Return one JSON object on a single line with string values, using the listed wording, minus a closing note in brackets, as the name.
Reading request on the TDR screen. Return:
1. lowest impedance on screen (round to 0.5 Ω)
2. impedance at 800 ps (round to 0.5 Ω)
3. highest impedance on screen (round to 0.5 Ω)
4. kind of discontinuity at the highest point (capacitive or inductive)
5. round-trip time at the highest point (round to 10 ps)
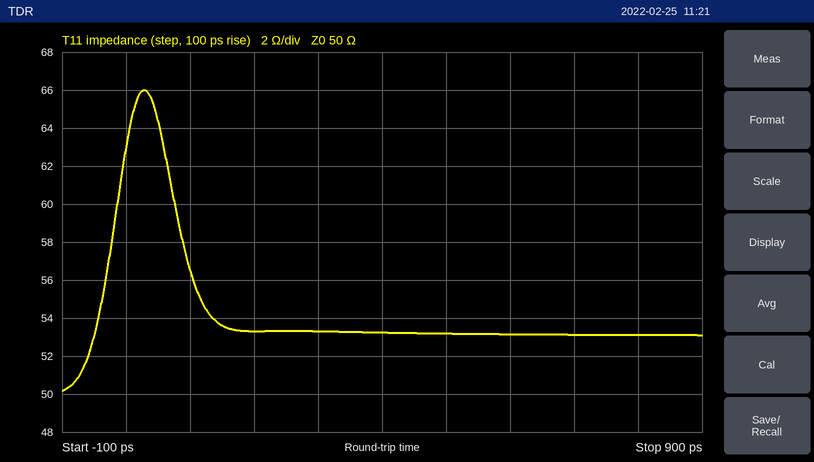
{"lowest impedance on screen": "50.0 Ω", "impedance at 800 ps": "53.0 Ω", "highest impedance on screen": "66.0 Ω", "kind of discontinuity at the highest point": "inductive", "round-trip time at the highest point": "30 ps"}
